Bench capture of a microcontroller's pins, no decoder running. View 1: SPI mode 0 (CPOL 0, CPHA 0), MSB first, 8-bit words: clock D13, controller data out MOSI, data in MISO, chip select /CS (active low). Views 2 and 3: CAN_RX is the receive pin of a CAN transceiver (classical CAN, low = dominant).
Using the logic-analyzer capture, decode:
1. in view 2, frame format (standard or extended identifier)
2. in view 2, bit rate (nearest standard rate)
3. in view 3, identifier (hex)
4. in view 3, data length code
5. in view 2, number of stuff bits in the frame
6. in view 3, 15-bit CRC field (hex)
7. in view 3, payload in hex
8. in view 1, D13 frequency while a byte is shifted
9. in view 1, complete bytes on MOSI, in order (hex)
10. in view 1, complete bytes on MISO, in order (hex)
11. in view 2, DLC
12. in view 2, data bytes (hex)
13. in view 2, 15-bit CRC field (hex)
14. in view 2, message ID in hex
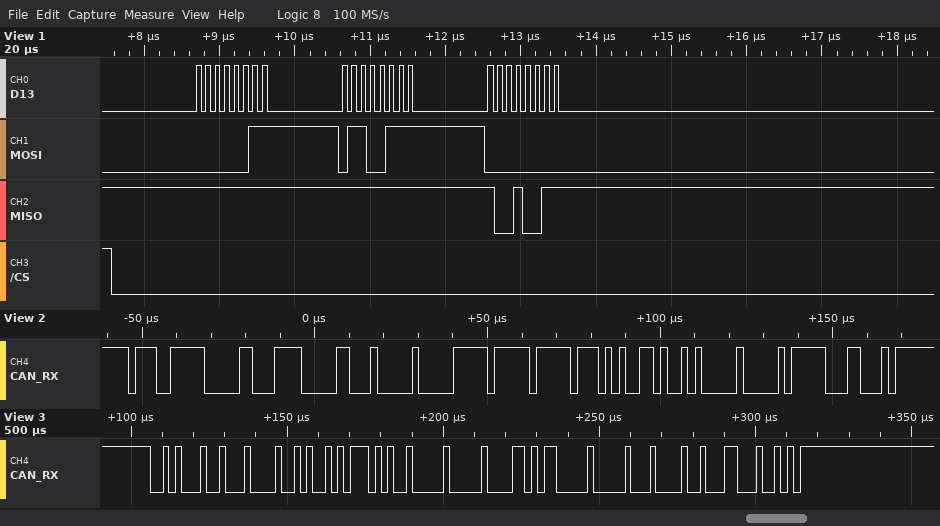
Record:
standard
500 kbit/s
0x289
8
11
0x2312
4A 57 52 00 06 B0 00 42
8 MHz
03 67 00
FF FF 93
8
F0 44 00 FF FF A9 A5 00
0x0F98
0x73E
